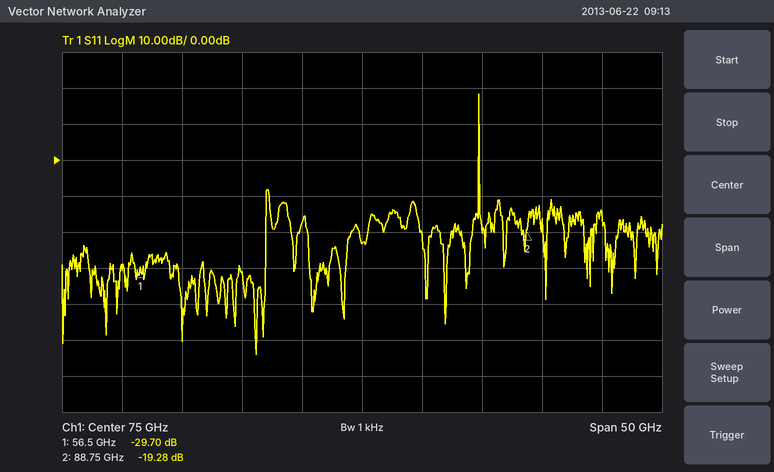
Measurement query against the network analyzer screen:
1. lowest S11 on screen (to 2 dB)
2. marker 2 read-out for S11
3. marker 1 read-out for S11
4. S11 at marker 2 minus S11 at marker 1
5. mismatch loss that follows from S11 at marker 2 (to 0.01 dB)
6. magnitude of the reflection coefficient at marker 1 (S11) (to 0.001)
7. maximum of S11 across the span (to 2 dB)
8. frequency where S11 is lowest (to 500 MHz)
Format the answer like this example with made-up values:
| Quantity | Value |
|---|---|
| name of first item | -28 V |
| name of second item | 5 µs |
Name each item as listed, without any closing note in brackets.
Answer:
| Quantity | Value |
|---|---|
| lowest S11 on screen | -54 dB |
| marker 2 read-out for S11 | -19.28 dB |
| marker 1 read-out for S11 | -29.70 dB |
| S11 at marker 2 minus S11 at marker 1 | 10.42 dB |
| mismatch loss that follows from S11 at marker 2 | 0.05 dB |
| magnitude of the reflection coefficient at marker 1 (S11) | 0.033 |
| maximum of S11 across the span | 18 dB |
| frequency where S11 is lowest | 66.0 GHz |
